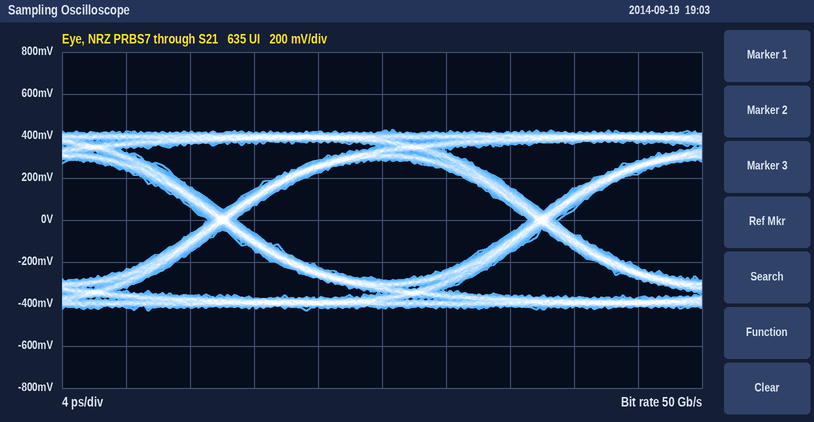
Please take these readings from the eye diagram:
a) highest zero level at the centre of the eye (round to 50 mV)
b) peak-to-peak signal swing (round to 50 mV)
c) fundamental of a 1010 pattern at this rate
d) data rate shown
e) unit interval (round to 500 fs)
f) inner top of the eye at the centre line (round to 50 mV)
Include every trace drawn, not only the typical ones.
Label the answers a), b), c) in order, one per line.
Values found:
a) -300 mV
b) 850 mV
c) 25 GHz
d) 50 Gb/s
e) 20.0 ps
f) 300 mV
